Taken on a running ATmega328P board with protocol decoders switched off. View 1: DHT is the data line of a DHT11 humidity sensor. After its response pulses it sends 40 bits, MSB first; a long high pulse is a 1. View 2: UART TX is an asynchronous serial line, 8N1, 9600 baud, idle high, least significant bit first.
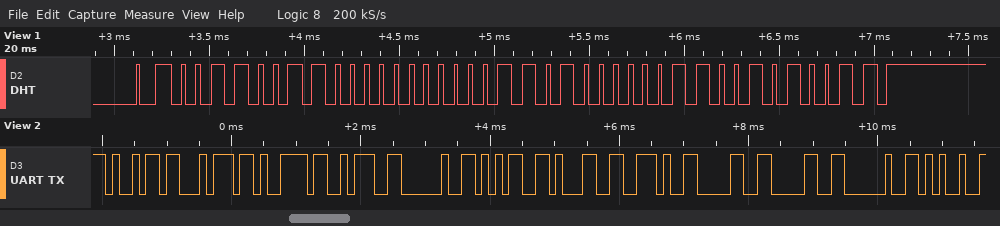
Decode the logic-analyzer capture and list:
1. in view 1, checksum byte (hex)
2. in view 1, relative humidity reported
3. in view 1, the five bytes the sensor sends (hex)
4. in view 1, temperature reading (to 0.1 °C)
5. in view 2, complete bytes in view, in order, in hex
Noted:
0x53
51 %
33 00 1A 06 53
26.6 °C
69 74 79 3A 20 35 31 2E 30 30 20 25
